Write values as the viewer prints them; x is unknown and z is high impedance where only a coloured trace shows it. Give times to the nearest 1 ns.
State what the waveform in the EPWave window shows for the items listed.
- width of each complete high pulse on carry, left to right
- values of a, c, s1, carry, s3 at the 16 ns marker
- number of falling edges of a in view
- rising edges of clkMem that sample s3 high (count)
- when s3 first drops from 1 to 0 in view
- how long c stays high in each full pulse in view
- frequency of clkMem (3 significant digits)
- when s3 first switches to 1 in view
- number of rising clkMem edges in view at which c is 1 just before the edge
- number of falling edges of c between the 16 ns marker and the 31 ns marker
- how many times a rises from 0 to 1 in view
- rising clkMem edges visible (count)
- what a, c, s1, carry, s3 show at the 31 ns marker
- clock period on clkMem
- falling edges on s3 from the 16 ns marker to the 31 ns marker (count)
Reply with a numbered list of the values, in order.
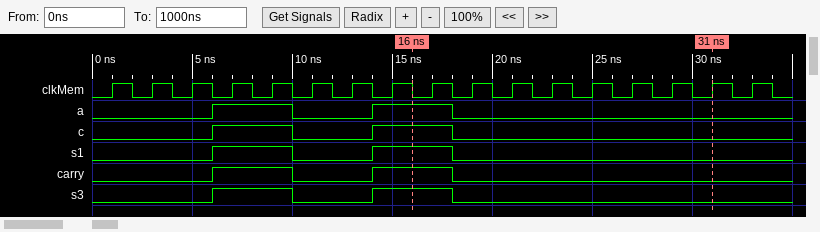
1. 4 ns, 4 ns
2. a=1, c=1, s1=1, carry=1, s3=1
3. 2
4. 4
5. 10 ns
6. 4 ns, 4 ns
7. 500 MHz
8. 6 ns
9. 4
10. 1
11. 2
12. 17
13. a=0, c=0, s1=0, carry=0, s3=0
14. 2 ns
15. 1
